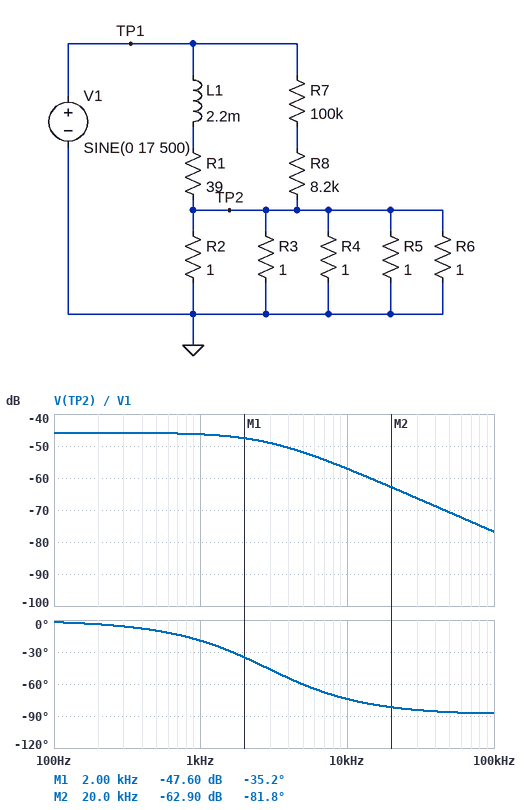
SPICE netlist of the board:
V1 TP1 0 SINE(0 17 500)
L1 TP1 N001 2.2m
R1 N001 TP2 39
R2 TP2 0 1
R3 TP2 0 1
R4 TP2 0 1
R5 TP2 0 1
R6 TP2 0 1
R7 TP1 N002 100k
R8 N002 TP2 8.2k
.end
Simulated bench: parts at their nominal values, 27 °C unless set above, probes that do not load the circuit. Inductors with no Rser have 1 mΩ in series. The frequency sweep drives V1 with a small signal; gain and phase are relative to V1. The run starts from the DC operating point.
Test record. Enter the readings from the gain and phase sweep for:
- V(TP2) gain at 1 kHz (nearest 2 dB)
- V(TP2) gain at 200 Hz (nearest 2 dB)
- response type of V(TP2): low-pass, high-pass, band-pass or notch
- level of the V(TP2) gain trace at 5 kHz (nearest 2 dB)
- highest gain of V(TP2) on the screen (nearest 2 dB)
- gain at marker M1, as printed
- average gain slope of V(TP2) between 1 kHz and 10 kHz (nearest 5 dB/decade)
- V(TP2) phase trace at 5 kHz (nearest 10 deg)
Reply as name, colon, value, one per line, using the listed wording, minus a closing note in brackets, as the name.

V(TP2) gain at 1 kHz: -46 dB
V(TP2) gain at 200 Hz: -46 dB
response type of V(TP2): low-pass, high-pass, band-pass or notch: low-pass
level of the V(TP2) gain trace at 5 kHz: -52 dB
highest gain of V(TP2) on the screen: -46 dB
gain at marker M1, as printed: -47.60 dB
average gain slope of V(TP2) between 1 kHz and 10 kHz: -10 dB/decade
V(TP2) phase trace at 5 kHz: -60 deg
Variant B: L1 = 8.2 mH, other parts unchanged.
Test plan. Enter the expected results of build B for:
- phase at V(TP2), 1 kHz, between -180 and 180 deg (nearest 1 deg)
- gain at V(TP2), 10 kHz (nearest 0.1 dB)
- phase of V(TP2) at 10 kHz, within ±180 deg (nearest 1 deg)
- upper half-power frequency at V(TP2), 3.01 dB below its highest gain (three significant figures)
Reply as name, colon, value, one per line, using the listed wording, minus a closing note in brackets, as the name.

phase at V(TP2), 1 kHz, between -180 and 180 deg: -53 deg
gain at V(TP2), 10 kHz: -68.2 dB
phase of V(TP2) at 10 kHz, within ±180 deg: -85 deg
upper half-power frequency at V(TP2), 3.01 dB below its highest gain: 761 Hz
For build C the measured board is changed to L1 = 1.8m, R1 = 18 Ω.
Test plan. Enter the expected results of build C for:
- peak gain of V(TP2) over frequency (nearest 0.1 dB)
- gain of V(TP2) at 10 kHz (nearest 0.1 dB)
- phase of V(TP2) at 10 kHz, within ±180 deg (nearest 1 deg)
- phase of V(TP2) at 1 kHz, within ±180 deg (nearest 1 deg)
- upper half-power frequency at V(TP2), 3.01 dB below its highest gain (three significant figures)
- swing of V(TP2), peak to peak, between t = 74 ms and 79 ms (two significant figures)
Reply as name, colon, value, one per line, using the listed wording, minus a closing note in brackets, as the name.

peak gain of V(TP2) over frequency: -39.2 dB
gain of V(TP2) at 10 kHz: -55.2 dB
phase of V(TP2) at 10 kHz, within ±180 deg: -81 deg
phase of V(TP2) at 1 kHz, within ±180 deg: -32 deg
upper half-power frequency at V(TP2), 3.01 dB below its highest gain: 1.61 kHz
swing of V(TP2), peak to peak, between t = 74 ms and 79 ms: 360 mV
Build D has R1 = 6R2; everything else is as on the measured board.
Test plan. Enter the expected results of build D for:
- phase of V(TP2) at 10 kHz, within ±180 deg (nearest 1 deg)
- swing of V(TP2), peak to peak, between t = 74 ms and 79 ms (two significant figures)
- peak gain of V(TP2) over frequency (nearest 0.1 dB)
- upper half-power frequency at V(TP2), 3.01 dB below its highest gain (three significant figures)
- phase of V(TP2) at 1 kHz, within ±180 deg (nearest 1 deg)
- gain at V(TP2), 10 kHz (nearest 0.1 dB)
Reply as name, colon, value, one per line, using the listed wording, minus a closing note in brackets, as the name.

phase of V(TP2) at 10 kHz, within ±180 deg: -87 deg
swing of V(TP2), peak to peak, between t = 74 ms and 79 ms: 720 mV
peak gain of V(TP2) over frequency: -30.1 dB
upper half-power frequency at V(TP2), 3.01 dB below its highest gain: 463 Hz
phase of V(TP2) at 1 kHz, within ±180 deg: -65 deg
gain at V(TP2), 10 kHz: -56.8 dB
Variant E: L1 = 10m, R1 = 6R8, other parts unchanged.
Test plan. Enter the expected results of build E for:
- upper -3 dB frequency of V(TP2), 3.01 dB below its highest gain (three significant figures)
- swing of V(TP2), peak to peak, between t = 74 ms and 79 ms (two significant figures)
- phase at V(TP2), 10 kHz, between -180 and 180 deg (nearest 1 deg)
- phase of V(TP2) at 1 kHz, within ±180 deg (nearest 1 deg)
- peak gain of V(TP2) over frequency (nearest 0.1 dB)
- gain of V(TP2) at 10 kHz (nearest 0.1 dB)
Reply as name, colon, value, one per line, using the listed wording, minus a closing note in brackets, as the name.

upper -3 dB frequency of V(TP2), 3.01 dB below its highest gain: 111 Hz
swing of V(TP2), peak to peak, between t = 74 ms and 79 ms: 210 mV
phase at V(TP2), 10 kHz, between -180 and 180 deg: -89 deg
phase of V(TP2) at 1 kHz, within ±180 deg: -84 deg
peak gain of V(TP2) over frequency: -30.9 dB
gain of V(TP2) at 10 kHz: -69.9 dB
